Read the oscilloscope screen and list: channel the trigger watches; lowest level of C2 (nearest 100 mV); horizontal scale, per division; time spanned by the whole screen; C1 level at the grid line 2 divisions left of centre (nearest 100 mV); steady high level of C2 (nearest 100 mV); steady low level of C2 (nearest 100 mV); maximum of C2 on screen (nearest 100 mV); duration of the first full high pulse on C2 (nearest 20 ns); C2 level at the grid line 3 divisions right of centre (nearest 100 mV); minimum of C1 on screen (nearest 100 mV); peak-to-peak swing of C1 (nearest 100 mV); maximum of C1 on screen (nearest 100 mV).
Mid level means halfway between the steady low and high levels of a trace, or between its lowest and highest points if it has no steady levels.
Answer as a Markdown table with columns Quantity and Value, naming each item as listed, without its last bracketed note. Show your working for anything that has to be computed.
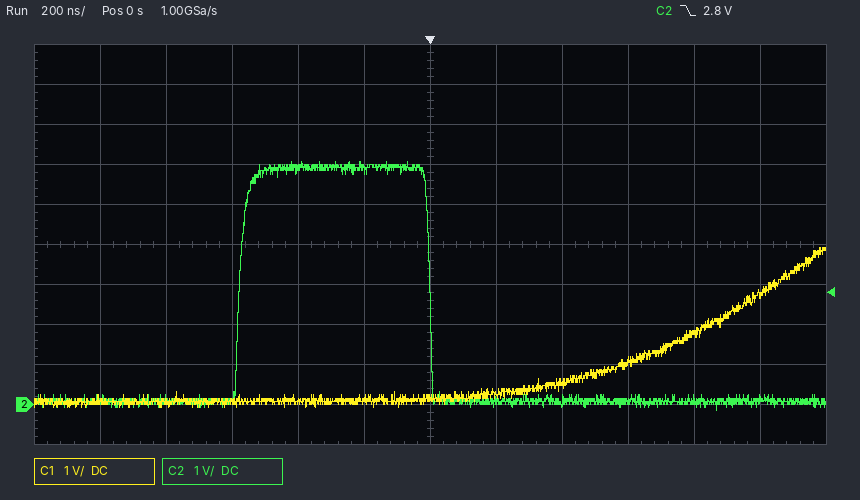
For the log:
| Quantity | Value |
|---|---|
| channel the trigger watches | C2 |
| lowest level of C2 | -200 mV |
| horizontal scale, per division | 200 ns |
| time spanned by the whole screen | 2.4 µs |
| C1 level at the grid line 2 divisions left of centre | 100 mV |
| steady high level of C2 | 5.9 V |
| steady low level of C2 | 100 mV |
| maximum of C2 on screen | 6.1 V |
| duration of the first full high pulse on C2 | 580 ns |
| C2 level at the grid line 3 divisions right of centre | 100 mV |
| minimum of C1 on screen | -100 mV |
| peak-to-peak swing of C1 | 3.9 V − (-100 mV) = 4.0 V |
| maximum of C1 on screen | 3.9 V |
